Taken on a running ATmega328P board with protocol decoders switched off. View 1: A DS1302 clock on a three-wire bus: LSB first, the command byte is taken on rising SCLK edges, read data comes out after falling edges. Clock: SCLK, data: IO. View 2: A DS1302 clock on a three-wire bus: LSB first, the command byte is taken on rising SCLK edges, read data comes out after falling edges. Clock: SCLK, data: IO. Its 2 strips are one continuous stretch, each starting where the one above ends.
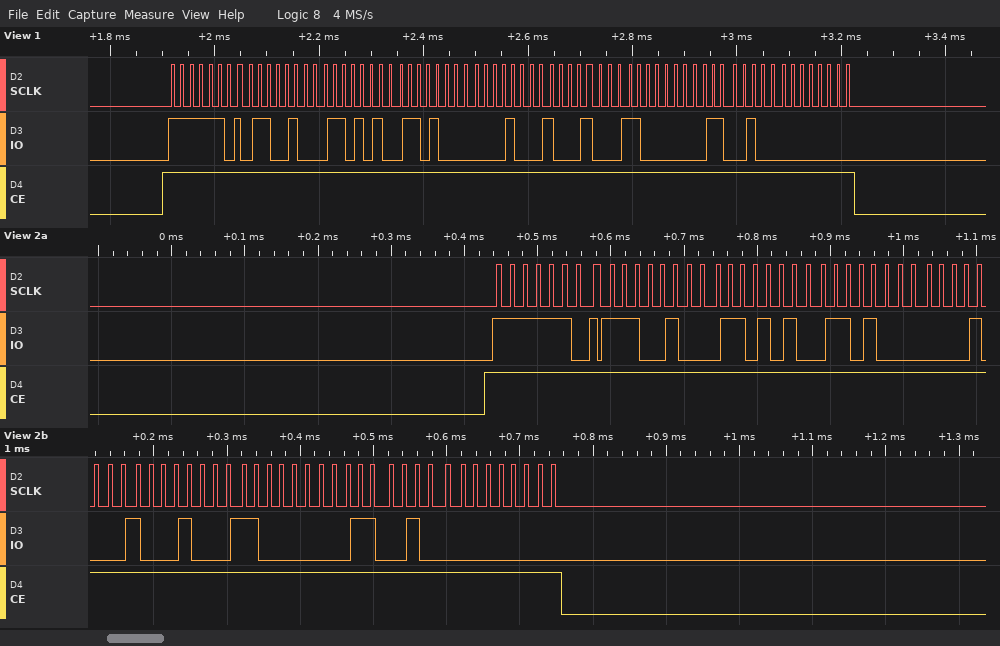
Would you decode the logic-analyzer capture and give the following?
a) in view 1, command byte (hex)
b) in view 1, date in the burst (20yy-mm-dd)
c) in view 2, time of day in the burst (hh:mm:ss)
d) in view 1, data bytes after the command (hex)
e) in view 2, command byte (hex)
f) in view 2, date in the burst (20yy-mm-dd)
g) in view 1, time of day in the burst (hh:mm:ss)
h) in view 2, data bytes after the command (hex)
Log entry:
0xBF
2026-11-10
16:56:27
26 56 16 10 11 03 26 00
0xBF
2026-11-10
16:56:26
27 56 16 10 11 03 26 00
